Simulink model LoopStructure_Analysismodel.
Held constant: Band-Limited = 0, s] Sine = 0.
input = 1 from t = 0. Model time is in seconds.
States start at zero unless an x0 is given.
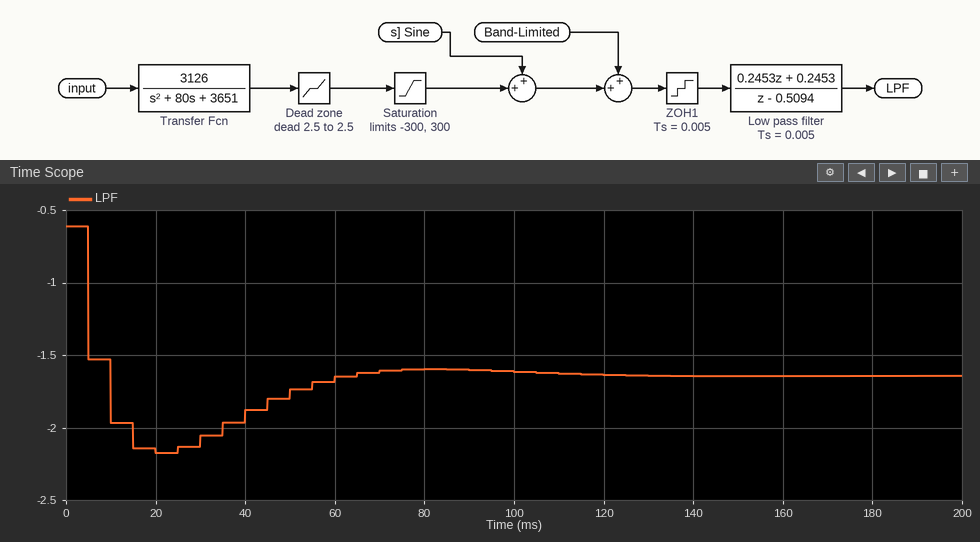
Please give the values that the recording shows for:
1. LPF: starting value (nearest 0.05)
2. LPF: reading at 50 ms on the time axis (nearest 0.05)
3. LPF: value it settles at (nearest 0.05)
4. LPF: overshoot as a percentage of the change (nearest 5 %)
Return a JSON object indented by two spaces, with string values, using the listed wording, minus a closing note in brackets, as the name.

{
  "LPF: starting value": "-0.60",
  "LPF: reading at 50 ms on the time axis": "-1.75",
  "LPF: value it settles at": "-1.65",
  "LPF: overshoot as a percentage of the change": "50 %"
}
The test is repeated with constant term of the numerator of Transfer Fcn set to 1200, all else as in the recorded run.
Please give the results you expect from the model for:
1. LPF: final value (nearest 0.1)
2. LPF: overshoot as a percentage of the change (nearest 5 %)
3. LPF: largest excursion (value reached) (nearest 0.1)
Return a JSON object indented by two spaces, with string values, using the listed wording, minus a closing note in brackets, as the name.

{
  "LPF: final value": "-2.2",
  "LPF: overshoot as a percentage of the change": "10 %",
  "LPF: largest excursion (value reached)": "-2.3"
}
